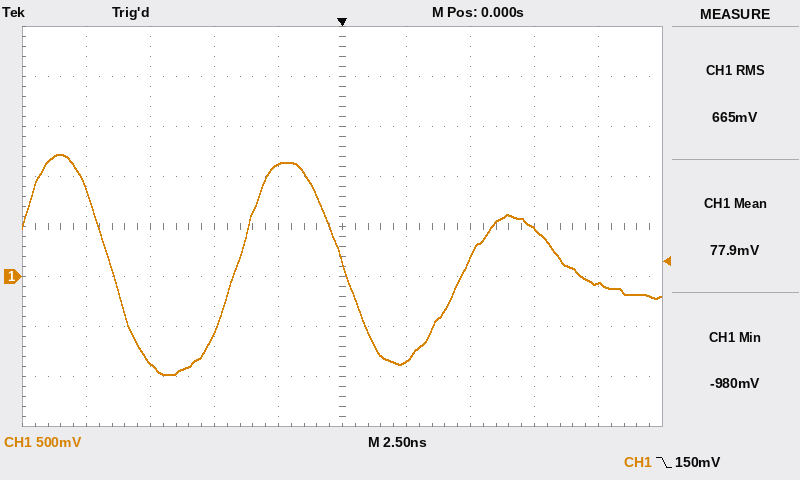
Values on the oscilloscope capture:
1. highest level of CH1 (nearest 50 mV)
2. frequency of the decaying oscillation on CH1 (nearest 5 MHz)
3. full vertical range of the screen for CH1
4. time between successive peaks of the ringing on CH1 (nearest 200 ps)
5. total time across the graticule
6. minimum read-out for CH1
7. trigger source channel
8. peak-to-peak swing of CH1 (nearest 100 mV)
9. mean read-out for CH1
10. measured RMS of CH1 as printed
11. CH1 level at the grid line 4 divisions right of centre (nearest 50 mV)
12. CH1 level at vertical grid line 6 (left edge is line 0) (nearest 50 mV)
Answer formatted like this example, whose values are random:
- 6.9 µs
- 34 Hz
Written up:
- 1.20 V
- 115 MHz
- 4 V
- 8.8 ns
- 25 ns
- -980 mV
- CH1
- 2.20 V
- 77.9 mV
- 665 mV
- -50 mV
- -850 mV
